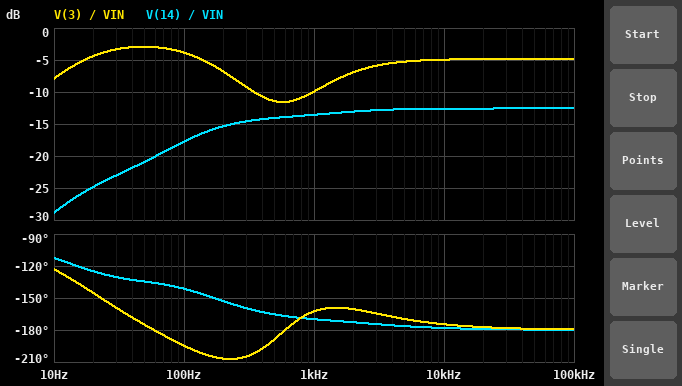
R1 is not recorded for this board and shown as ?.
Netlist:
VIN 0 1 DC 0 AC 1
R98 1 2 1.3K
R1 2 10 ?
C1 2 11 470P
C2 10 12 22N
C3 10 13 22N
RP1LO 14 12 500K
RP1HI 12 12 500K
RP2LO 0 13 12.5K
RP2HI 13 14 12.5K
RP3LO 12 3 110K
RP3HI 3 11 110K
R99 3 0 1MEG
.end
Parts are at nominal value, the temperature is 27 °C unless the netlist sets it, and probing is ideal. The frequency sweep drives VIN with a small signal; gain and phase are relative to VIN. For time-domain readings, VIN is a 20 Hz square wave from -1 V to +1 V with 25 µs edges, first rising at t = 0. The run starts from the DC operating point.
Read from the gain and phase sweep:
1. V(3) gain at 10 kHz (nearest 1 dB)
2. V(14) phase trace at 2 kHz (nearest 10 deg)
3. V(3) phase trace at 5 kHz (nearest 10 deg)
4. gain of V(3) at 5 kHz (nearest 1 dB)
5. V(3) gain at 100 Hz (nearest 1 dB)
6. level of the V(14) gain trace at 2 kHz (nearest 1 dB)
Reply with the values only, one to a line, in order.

-5 dB
-170 deg
-170 deg
-5 dB
-4 dB
-13 dB
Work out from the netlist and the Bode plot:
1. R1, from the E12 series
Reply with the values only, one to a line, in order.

47 kΩ
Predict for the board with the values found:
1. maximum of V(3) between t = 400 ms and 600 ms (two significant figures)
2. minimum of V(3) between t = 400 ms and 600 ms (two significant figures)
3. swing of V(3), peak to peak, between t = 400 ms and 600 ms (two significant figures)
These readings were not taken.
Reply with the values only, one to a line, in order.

1.1 V
-1.1 V
2.2 V
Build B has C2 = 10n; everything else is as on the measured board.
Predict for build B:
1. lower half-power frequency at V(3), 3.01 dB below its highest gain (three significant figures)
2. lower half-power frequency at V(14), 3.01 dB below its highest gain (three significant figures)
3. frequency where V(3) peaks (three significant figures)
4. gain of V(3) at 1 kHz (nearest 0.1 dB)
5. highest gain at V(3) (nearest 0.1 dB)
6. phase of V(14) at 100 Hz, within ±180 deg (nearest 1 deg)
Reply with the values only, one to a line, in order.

25.3 Hz
175 Hz
72.2 Hz
-9.7 dB
-3.8 dB
-140 deg
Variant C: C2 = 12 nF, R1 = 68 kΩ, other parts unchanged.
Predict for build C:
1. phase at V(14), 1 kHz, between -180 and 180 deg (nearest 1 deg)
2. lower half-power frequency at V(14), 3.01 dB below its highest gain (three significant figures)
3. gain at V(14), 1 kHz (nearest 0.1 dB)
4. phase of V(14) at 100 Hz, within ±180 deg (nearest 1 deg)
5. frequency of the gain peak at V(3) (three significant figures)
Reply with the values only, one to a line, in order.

-170 deg
172 Hz
-15.9 dB
-148 deg
56.5 Hz
